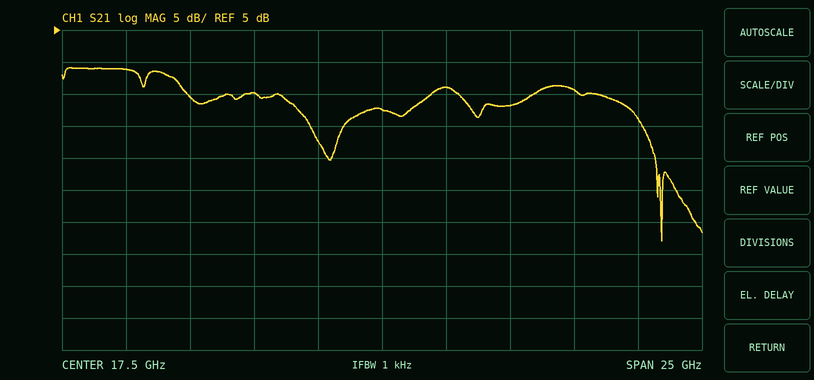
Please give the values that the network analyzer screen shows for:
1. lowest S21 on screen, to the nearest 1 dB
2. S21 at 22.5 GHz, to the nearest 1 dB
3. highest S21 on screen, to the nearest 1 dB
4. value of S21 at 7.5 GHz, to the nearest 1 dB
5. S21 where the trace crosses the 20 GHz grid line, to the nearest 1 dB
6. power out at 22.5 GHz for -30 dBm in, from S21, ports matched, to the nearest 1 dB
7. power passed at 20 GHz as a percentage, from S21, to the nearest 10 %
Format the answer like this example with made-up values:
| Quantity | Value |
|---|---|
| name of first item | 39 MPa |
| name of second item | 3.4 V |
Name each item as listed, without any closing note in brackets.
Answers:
| Quantity | Value |
|---|---|
| lowest S21 on screen, to the nearest 1 dB | -28 dB |
| S21 at 22.5 GHz, to the nearest 1 dB | -7 dB |
| highest S21 on screen, to the nearest 1 dB | -1 dB |
| value of S21 at 7.5 GHz, to the nearest 1 dB | -1 dB |
| S21 where the trace crosses the 20 GHz grid line, to the nearest 1 dB | -4 dB |
| power out at 22.5 GHz for -30 dBm in, from S21, ports matched, to the nearest 1 dB | -37 dBm |
| power passed at 20 GHz as a percentage, from S21, to the nearest 10 % | 40 % |
